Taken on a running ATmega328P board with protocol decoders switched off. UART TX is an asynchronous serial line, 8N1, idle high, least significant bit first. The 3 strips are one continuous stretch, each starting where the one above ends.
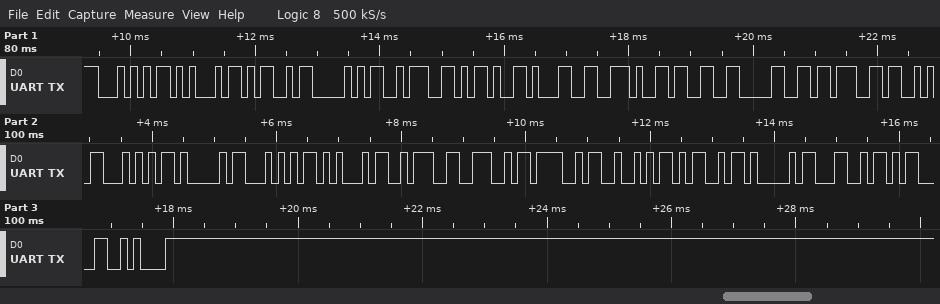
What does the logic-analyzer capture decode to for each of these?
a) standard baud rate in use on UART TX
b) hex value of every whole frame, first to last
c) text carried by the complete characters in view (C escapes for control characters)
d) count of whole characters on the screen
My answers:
9600 baud
54 45 4D 50 3A 2D 31 2E 33 30 3B 53 54 41 54 45 3A 4E 4F 52 4D 41 4C 0D 0A
"TEMP:-1.30;STATE:NORMAL\r\n"
25
